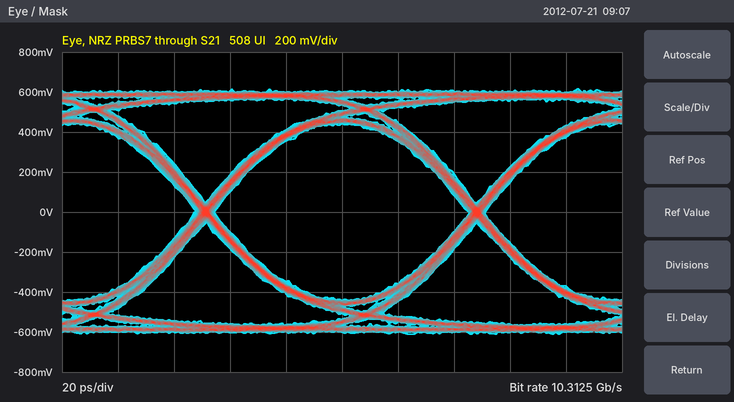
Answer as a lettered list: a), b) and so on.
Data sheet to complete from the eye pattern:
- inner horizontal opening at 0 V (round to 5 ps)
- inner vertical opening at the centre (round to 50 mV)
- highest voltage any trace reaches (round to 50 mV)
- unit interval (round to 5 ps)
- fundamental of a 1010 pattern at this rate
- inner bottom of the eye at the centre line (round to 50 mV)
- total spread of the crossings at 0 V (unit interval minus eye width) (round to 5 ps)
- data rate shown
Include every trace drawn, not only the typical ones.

a) 90 ps
b) 900 mV
c) 600 mV
d) 95 ps
e) 5.15625 GHz
f) -450 mV
g) 5 ps
h) 10.3125 Gb/s
